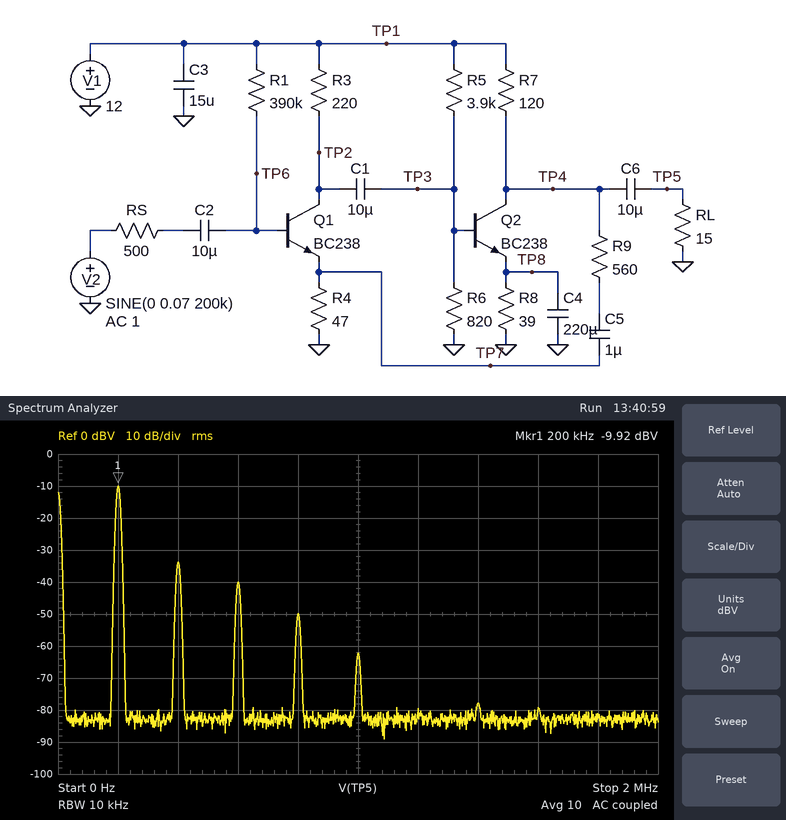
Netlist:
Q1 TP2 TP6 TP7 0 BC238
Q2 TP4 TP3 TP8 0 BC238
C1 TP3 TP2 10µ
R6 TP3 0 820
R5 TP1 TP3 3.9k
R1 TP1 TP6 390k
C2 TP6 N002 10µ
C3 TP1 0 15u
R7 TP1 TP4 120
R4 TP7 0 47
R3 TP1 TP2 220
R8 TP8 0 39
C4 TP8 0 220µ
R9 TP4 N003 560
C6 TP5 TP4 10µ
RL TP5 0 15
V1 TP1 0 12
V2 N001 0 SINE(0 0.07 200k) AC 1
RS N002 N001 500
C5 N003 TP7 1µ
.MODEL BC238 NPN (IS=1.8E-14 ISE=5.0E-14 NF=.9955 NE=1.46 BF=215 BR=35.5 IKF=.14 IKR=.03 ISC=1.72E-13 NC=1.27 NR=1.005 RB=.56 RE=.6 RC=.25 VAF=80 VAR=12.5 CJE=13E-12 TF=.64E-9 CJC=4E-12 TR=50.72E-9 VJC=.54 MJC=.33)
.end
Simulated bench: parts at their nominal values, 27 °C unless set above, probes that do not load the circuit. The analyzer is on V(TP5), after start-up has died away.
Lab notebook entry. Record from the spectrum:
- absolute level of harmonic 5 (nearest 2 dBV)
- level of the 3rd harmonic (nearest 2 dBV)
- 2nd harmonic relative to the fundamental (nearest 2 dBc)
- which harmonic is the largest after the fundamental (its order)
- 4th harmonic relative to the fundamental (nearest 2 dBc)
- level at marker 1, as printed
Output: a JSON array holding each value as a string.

["-62 dBV", "-40 dBV", "-24 dBc", "2", "-40 dBc", "-9.92 dBV"]
